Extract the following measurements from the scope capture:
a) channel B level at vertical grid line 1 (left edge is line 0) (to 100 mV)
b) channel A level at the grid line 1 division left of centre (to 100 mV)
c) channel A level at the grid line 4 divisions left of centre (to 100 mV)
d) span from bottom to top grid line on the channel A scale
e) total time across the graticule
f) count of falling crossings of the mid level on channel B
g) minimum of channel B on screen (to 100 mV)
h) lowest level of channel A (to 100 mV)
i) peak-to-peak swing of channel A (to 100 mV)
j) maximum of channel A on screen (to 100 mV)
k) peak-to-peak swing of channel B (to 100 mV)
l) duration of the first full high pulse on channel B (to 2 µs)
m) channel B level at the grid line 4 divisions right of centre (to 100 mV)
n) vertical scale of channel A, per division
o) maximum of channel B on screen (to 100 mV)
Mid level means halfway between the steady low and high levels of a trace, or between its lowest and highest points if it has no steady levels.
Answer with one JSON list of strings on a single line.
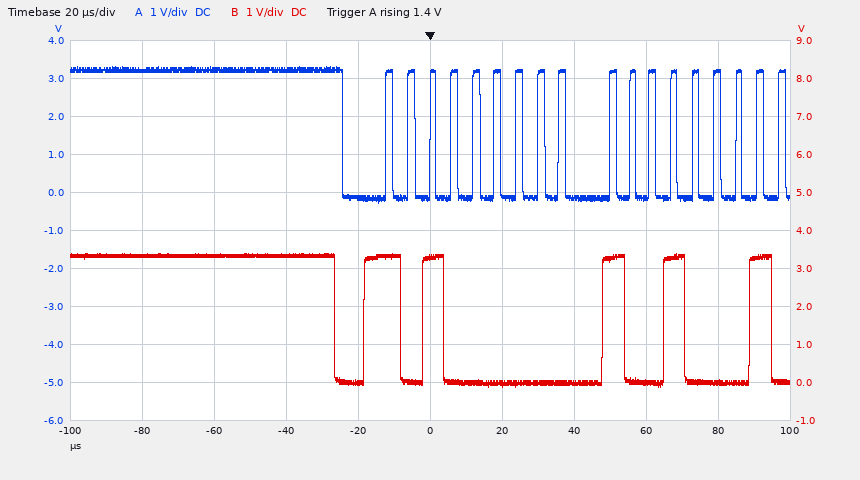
["3.3 V", "-100 mV", "3.2 V", "10 V", "200 µs", "6", "-100 mV", "-300 mV", "3.6 V", "3.3 V", "3.5 V", "10 µs", "0.0 V", "1 V", "3.4 V"]
